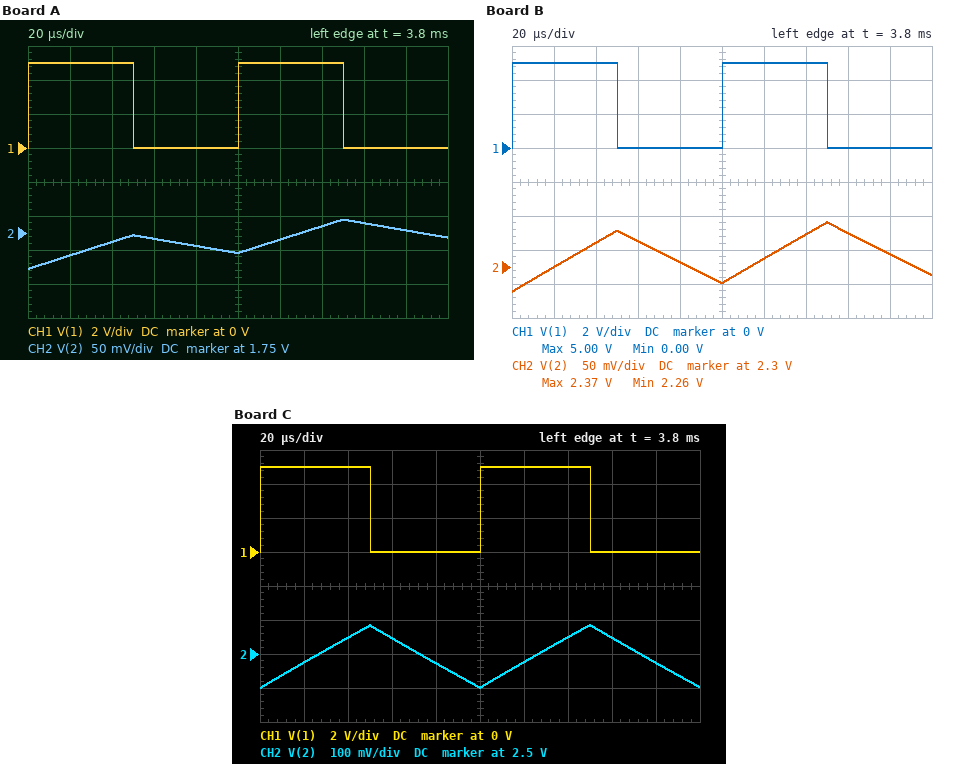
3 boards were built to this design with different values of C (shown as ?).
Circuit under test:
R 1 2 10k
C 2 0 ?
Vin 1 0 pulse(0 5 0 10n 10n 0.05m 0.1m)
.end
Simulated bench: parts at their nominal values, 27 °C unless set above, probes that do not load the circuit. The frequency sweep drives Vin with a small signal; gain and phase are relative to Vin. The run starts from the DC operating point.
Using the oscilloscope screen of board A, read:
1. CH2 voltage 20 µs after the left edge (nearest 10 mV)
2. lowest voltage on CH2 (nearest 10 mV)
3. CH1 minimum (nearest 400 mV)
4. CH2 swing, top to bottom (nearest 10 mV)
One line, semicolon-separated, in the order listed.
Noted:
1.72 V; 1.70 V; 0 V; 70 mV
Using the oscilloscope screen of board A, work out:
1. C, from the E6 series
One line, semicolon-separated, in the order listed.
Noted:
330 nF
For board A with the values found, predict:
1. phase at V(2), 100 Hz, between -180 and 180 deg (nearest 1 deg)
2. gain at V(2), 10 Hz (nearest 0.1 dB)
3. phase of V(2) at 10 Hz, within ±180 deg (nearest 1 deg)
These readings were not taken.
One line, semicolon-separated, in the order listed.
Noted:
-64 deg; -0.2 dB; -12 deg
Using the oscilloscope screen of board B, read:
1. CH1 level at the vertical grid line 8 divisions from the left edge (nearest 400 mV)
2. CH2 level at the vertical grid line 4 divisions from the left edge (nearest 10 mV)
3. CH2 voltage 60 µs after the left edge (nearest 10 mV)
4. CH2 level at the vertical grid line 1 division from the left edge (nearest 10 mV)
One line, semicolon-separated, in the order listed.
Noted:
0 V; 2.31 V; 2.34 V; 2.30 V
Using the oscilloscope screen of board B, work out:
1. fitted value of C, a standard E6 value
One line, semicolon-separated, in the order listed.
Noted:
150 nF
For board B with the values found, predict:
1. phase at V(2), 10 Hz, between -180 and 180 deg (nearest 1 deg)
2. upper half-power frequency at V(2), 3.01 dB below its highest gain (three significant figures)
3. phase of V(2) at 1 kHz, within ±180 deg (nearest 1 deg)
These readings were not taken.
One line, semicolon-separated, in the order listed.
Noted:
-5 deg; 106 Hz; -84 deg
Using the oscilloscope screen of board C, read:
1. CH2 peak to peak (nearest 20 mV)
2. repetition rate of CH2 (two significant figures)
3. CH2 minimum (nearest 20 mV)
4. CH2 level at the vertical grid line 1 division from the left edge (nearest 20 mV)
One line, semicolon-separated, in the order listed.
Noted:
180 mV; 10 kHz; 2.40 V; 2.48 V
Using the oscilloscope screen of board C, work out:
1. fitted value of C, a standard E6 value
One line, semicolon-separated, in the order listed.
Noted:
68 nF
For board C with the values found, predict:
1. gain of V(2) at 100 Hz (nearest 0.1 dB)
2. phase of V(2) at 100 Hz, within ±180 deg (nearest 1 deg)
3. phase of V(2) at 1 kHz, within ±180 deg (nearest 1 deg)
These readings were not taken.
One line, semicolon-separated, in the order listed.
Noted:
-0.7 dB; -23 deg; -77 deg
